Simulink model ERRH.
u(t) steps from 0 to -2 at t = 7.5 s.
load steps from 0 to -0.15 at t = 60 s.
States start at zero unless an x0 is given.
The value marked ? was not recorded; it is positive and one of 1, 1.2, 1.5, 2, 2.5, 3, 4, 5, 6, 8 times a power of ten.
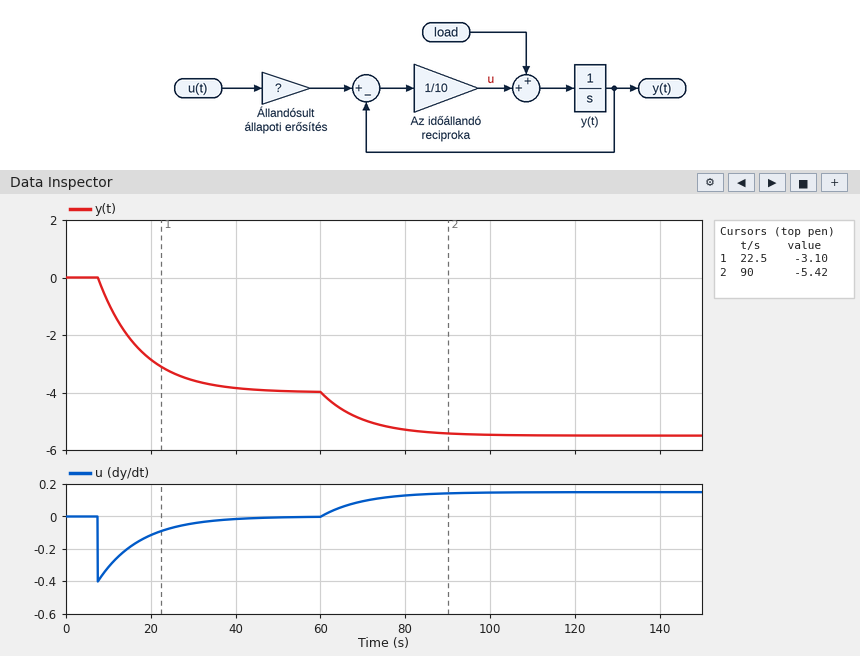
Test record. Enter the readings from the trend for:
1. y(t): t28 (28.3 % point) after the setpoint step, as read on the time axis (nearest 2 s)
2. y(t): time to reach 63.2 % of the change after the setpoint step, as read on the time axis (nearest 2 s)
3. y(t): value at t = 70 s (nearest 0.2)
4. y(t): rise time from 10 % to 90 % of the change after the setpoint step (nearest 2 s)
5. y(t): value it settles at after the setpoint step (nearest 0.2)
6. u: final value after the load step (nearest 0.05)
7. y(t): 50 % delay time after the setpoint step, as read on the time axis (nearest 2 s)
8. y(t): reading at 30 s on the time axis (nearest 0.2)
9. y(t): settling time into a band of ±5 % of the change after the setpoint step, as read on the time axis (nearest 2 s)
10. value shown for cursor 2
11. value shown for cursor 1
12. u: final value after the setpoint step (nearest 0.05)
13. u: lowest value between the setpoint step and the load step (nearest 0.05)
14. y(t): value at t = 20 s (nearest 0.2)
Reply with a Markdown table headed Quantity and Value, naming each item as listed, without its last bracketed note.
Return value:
| Quantity | Value |
|---|---|
| y(t): t28 (28.3 % point) after the setpoint step, as read on the time axis | 10 s |
| y(t): time to reach 63.2 % of the change after the setpoint step, as read on the time axis | 18 s |
| y(t): value at t = 70 s | -5.0 |
| y(t): rise time from 10 % to 90 % of the change after the setpoint step | 22 s |
| y(t): value it settles at after the setpoint step | -4.0 |
| u: final value after the load step | 0.15 |
| y(t): 50 % delay time after the setpoint step, as read on the time axis | 14 s |
| y(t): reading at 30 s on the time axis | -3.6 |
| y(t): settling time into a band of ±5 % of the change after the setpoint step, as read on the time axis | 38 s |
| value shown for cursor 2 | -5.42 |
| value shown for cursor 1 | -3.10 |
| u: final value after the setpoint step | 0.00 |
| u: lowest value between the setpoint step and the load step | -0.40 |
| y(t): value at t = 20 s | -2.8 |
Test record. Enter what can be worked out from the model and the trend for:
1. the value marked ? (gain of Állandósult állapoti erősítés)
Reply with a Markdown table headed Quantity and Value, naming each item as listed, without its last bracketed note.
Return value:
| Quantity | Value |
|---|---|
| the value marked ? | 2 |
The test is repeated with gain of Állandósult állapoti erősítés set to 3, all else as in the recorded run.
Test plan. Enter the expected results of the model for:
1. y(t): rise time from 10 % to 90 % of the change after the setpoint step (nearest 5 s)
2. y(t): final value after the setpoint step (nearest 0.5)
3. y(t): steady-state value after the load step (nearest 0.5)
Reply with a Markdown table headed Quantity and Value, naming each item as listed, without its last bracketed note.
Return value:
| Quantity | Value |
|---|---|
| y(t): rise time from 10 % to 90 % of the change after the setpoint step | 20 s |
| y(t): final value after the setpoint step | -6.0 |
| y(t): steady-state value after the load step | -7.5 |
